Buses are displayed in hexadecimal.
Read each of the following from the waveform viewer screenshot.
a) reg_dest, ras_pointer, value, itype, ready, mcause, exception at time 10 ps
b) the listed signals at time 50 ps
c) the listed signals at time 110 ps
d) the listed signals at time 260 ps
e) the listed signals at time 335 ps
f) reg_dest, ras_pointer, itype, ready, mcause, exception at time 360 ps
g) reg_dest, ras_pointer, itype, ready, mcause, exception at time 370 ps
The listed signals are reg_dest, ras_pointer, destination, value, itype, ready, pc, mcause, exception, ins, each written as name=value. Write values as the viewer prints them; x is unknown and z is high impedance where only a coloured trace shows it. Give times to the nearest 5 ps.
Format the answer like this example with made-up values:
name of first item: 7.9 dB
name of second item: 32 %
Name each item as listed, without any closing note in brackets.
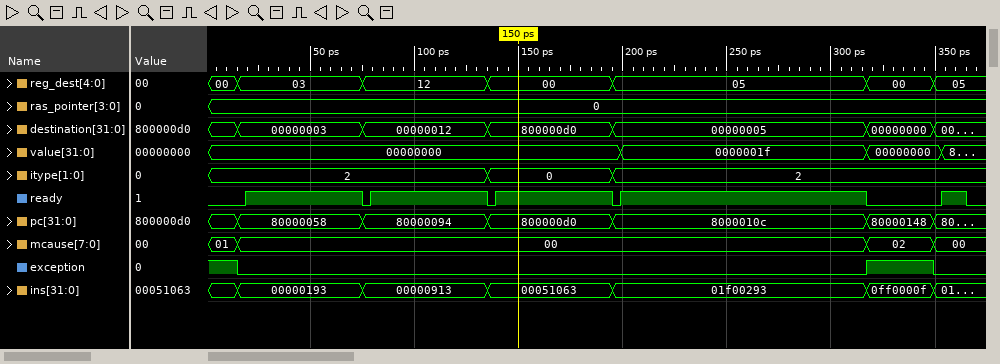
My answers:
reg_dest, ras_pointer, value, itype, ready, mcause, exception at time 10 ps: reg_dest=00, ras_pointer=0, value=00000000, itype=2, ready=0, mcause=01, exception=1
the listed signals at time 50 ps: reg_dest=03, ras_pointer=0, destination=00000003, value=00000000, itype=2, ready=1, pc=80000058, mcause=00, exception=0, ins=00000193
the listed signals at time 110 ps: reg_dest=12, ras_pointer=0, destination=00000012, value=00000000, itype=2, ready=1, pc=80000094, mcause=00, exception=0, ins=00000913
the listed signals at time 260 ps: reg_dest=05, ras_pointer=0, destination=00000005, value=0000001f, itype=2, ready=1, pc=8000010c, mcause=00, exception=0, ins=01f00293
the listed signals at time 335 ps: reg_dest=00, ras_pointer=0, destination=00000000, value=00000000, itype=2, ready=0, pc=80000148, mcause=02, exception=1, ins=0ff0000f
reg_dest, ras_pointer, itype, ready, mcause, exception at time 360 ps: reg_dest=05, ras_pointer=0, itype=2, ready=1, mcause=00, exception=0
reg_dest, ras_pointer, itype, ready, mcause, exception at time 370 ps: reg_dest=05, ras_pointer=0, itype=2, ready=0, mcause=00, exception=0
